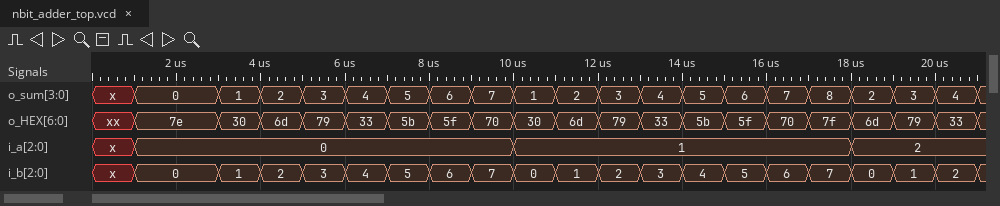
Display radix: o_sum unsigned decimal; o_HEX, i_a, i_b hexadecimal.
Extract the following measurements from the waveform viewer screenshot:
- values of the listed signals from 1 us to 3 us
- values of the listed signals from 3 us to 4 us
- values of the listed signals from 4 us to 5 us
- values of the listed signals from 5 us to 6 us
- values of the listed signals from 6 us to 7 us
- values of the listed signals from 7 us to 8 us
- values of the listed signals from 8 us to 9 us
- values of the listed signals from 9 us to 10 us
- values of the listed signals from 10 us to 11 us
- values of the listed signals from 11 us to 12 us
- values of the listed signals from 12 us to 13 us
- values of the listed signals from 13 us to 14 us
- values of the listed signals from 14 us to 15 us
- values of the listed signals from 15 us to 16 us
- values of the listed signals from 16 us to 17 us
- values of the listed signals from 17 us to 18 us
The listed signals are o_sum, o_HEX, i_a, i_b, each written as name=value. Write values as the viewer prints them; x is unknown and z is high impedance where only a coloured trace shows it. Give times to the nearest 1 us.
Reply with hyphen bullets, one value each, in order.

- o_sum=0, o_HEX=7e, i_a=0, i_b=0
- o_sum=1, o_HEX=30, i_a=0, i_b=1
- o_sum=2, o_HEX=6d, i_a=0, i_b=2
- o_sum=3, o_HEX=79, i_a=0, i_b=3
- o_sum=4, o_HEX=33, i_a=0, i_b=4
- o_sum=5, o_HEX=5b, i_a=0, i_b=5
- o_sum=6, o_HEX=5f, i_a=0, i_b=6
- o_sum=7, o_HEX=70, i_a=0, i_b=7
- o_sum=1, o_HEX=30, i_a=1, i_b=0
- o_sum=2, o_HEX=6d, i_a=1, i_b=1
- o_sum=3, o_HEX=79, i_a=1, i_b=2
- o_sum=4, o_HEX=33, i_a=1, i_b=3
- o_sum=5, o_HEX=5b, i_a=1, i_b=4
- o_sum=6, o_HEX=5f, i_a=1, i_b=5
- o_sum=7, o_HEX=70, i_a=1, i_b=6
- o_sum=8, o_HEX=7f, i_a=1, i_b=7
